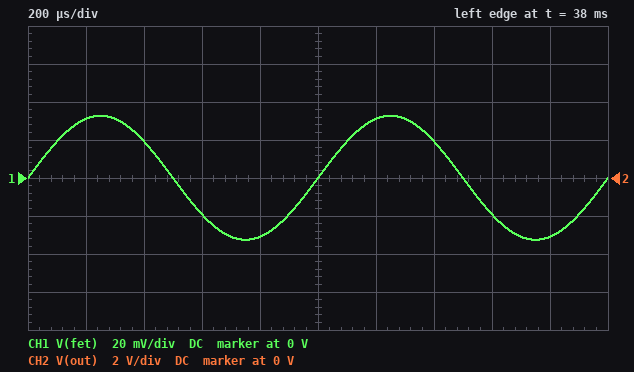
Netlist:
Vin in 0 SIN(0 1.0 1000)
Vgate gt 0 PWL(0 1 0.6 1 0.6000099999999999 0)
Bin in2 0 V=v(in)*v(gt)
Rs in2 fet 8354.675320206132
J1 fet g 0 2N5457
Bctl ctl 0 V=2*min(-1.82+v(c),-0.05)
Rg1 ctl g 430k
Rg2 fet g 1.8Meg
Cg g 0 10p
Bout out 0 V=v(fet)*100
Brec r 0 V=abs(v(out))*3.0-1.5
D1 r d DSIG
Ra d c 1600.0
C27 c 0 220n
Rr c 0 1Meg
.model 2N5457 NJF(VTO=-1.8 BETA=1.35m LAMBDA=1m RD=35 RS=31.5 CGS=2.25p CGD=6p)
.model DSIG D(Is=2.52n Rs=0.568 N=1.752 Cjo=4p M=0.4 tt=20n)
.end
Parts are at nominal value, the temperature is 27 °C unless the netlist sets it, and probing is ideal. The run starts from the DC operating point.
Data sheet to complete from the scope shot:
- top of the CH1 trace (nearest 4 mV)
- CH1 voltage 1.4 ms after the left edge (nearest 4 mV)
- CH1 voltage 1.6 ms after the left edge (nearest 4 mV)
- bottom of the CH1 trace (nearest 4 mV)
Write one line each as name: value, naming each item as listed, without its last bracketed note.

top of the CH1 trace: 32 mV
CH1 voltage 1.4 ms after the left edge: 20 mV
CH1 voltage 1.6 ms after the left edge: -20 mV
bottom of the CH1 trace: -32 mV
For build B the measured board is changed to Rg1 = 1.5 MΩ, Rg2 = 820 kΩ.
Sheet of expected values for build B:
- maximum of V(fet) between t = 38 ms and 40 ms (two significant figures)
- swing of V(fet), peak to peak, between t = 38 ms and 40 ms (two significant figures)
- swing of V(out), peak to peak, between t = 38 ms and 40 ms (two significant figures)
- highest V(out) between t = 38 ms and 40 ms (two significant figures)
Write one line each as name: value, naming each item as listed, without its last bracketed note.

maximum of V(fet) between t = 38 ms and 40 ms: 32 mV
swing of V(fet), peak to peak, between t = 38 ms and 40 ms: 64 mV
swing of V(out), peak to peak, between t = 38 ms and 40 ms: 6.4 V
highest V(out) between t = 38 ms and 40 ms: 3.2 V
